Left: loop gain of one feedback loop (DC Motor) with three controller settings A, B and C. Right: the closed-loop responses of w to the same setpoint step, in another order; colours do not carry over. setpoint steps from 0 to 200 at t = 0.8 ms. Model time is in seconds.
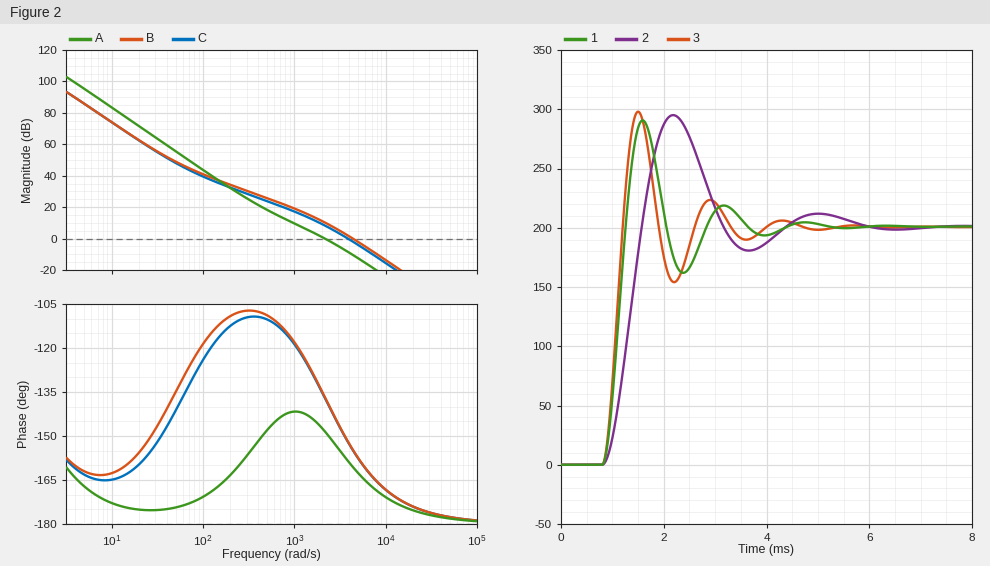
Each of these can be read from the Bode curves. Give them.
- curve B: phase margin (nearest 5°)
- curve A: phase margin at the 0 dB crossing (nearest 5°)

25°
30°
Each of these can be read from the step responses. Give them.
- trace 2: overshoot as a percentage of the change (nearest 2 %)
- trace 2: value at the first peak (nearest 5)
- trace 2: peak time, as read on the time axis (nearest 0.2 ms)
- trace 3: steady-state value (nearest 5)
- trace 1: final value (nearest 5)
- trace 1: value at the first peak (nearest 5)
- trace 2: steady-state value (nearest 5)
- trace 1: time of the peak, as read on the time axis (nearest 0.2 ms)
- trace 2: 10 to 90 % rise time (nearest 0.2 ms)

48 %
295
2.2 ms
200
200
290
200
1.6 ms
0.6 ms
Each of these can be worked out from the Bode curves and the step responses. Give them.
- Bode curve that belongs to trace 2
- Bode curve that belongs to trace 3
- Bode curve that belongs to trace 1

A
B
C
